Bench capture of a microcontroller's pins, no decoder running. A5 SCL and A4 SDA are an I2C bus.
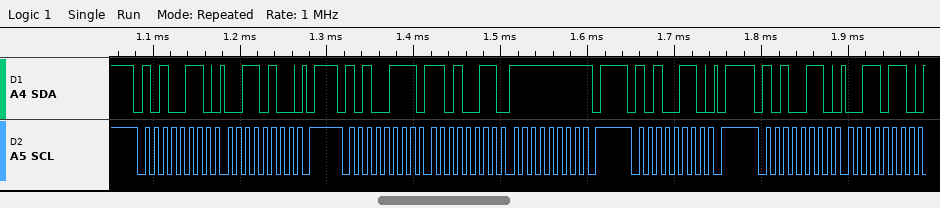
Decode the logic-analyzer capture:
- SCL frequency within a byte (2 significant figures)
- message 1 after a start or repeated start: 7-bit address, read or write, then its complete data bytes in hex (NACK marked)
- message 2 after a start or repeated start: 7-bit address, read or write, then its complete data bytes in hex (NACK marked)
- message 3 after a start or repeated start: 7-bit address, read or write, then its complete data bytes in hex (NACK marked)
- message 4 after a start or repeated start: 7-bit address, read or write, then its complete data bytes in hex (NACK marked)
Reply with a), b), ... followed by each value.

a) 100 kHz
b) 0x53 write: 34
c) 0x53 read: D3 FF NACK
d) 0x53 write
e) 0x53 write: 36
